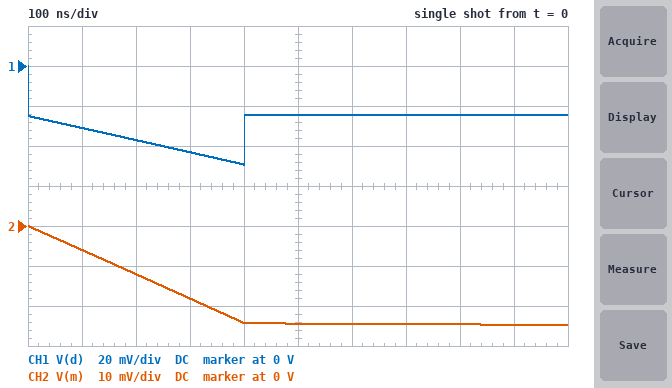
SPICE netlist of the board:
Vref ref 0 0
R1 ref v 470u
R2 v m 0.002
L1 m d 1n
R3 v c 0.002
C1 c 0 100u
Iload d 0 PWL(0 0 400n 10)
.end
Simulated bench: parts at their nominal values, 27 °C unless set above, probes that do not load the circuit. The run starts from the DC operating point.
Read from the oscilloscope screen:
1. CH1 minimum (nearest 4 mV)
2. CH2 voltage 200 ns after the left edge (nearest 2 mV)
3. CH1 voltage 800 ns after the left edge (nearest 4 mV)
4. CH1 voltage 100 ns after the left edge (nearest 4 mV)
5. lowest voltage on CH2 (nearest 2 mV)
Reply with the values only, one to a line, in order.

-48 mV
-12 mV
-24 mV
-32 mV
-24 mV
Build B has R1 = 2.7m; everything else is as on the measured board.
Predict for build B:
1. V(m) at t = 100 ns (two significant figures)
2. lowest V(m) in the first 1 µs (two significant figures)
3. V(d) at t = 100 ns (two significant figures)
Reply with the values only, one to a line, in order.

-8.3 mV
-44 mV
-33 mV
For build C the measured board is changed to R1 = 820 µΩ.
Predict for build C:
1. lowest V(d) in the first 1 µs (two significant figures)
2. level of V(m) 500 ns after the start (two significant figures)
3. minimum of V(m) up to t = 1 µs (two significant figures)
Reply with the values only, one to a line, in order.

-52 mV
-27 mV
-28 mV
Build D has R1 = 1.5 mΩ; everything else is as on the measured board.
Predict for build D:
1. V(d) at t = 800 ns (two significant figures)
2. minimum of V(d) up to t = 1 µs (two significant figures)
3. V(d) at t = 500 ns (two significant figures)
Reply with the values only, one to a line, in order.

-34 mV
-56 mV
-32 mV
